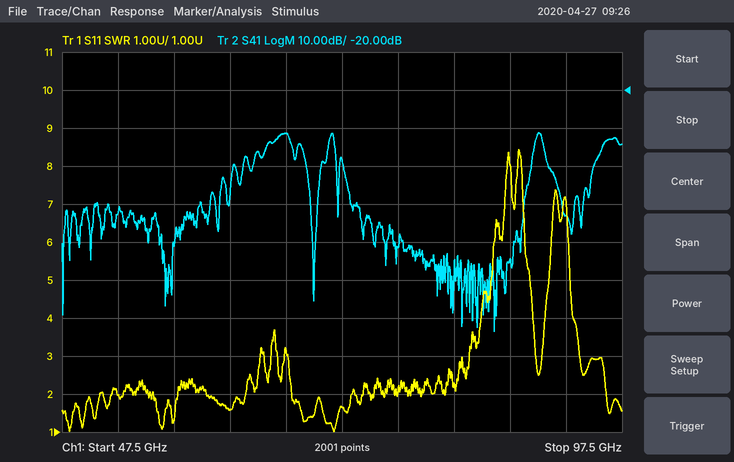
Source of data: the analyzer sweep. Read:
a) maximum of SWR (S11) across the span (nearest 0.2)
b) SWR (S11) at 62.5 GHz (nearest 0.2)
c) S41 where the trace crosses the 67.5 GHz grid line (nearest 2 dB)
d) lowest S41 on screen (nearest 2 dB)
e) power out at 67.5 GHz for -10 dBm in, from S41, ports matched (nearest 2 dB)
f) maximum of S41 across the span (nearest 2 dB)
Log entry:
8.4
1.6
-32 dB
-84 dB
-42 dBm
-32 dB
